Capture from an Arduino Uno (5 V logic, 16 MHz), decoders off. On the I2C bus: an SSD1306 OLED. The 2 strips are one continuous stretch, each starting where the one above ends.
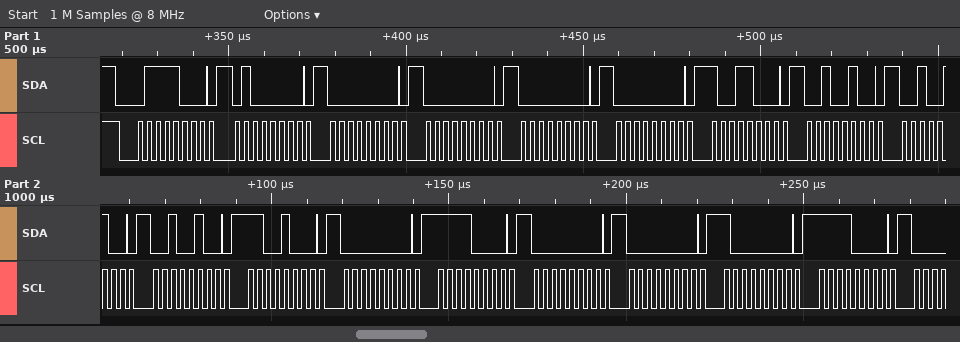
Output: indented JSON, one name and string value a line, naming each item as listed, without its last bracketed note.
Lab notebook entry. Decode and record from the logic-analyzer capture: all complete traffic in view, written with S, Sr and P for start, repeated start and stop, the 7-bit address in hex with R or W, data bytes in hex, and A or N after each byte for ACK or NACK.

{
  "all complete traffic in view, written with S, Sr and P for start, repeated start and stop, the 7-bit address in hex with R or W, data bytes in hex, and A or N after each byte for ACK or NACK": "S 3CW A 40 A 00 A 00 A 00 A 00 A 98 A 24 A 24 A 24 A C8 A 00 A F0 A 00 A 00 A 80 A F0 A"
}
